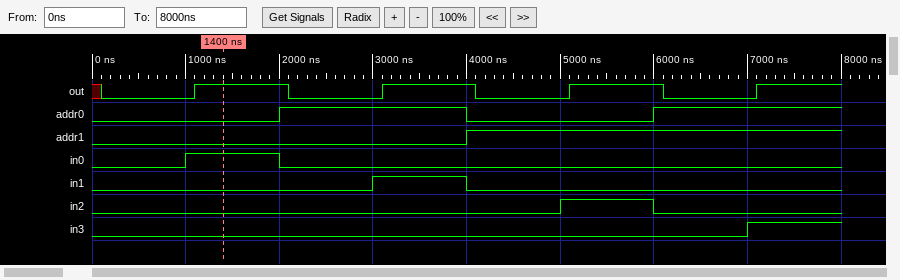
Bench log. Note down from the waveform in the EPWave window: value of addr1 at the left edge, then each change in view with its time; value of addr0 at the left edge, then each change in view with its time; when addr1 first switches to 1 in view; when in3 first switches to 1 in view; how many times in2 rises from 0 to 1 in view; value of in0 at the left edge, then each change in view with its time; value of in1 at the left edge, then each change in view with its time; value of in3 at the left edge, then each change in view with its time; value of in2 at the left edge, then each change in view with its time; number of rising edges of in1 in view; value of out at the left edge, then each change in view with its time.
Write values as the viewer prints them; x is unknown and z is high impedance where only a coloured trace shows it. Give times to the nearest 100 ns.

0, 1 at 4000 ns
0, 1 at 2000 ns, 0 at 4000 ns, 1 at 6000 ns
4000 ns
7000 ns
1
0, 1 at 1000 ns, 0 at 2000 ns
0, 1 at 3000 ns, 0 at 4000 ns
0, 1 at 7000 ns
0, 1 at 5000 ns, 0 at 6000 ns
1
x, 0 at 100 ns, 1 at 1100 ns, 0 at 2100 ns, 1 at 3100 ns, 0 at 4100 ns, 1 at 5100 ns, 0 at 6100 ns, 1 at 7100 ns
